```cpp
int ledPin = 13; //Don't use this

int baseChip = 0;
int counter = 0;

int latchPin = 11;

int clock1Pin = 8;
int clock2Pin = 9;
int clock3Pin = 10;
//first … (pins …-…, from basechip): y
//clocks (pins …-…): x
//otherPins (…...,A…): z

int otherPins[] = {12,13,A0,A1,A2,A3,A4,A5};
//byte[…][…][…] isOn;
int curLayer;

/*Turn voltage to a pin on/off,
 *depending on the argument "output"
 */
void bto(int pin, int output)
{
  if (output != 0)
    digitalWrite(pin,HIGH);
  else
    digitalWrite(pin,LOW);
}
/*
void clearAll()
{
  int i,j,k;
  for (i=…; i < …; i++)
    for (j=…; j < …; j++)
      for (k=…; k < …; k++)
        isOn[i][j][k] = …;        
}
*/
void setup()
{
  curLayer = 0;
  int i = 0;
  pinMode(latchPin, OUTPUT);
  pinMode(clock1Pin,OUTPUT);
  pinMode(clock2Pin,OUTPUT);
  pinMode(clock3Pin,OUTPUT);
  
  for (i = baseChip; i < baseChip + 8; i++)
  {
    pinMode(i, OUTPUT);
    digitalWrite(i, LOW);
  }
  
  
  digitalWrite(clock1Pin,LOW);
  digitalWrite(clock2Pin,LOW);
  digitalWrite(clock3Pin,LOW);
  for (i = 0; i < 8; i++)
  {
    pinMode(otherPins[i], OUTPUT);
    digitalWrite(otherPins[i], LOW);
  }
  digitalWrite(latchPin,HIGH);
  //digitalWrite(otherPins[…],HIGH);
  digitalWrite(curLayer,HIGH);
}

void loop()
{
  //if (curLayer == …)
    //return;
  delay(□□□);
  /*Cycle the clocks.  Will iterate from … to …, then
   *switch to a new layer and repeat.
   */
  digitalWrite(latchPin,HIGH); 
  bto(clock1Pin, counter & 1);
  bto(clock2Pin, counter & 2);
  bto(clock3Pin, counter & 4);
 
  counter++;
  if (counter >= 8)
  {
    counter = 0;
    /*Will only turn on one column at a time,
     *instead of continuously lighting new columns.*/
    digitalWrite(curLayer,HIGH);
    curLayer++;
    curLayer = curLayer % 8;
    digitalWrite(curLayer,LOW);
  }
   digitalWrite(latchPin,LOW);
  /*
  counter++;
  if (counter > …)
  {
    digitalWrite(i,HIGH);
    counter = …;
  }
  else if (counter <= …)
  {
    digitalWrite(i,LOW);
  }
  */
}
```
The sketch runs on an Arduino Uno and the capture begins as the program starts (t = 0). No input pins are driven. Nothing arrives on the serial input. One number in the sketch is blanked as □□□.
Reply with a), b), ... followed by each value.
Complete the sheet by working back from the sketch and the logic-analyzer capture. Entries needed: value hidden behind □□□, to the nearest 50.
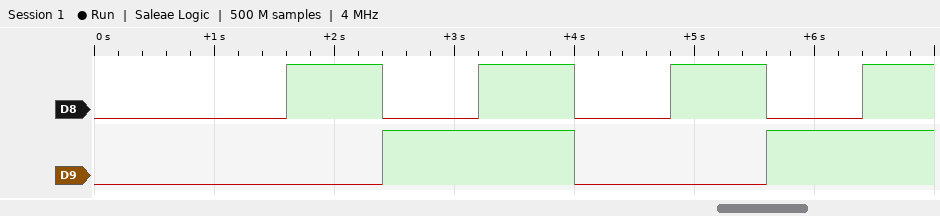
a) 800
